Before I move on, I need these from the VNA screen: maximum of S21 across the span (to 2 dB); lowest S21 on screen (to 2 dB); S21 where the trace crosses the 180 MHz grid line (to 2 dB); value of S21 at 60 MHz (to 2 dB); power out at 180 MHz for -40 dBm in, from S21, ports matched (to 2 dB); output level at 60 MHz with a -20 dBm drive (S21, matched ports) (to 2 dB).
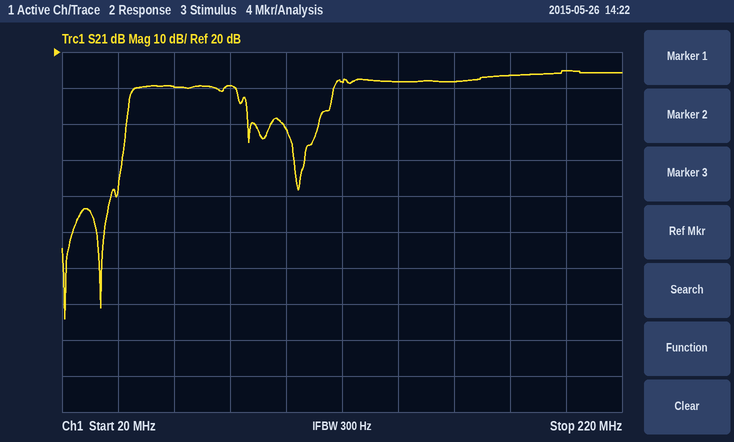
14 dB
-54 dB
14 dB
10 dB
-26 dBm
-10 dBm
